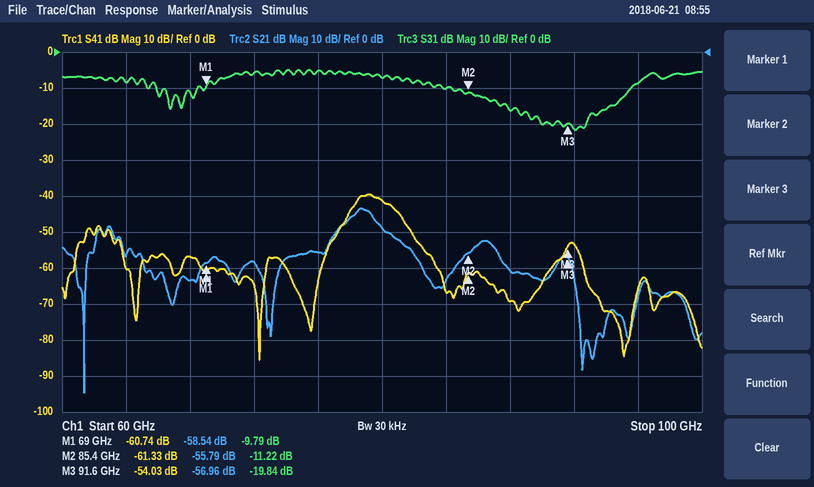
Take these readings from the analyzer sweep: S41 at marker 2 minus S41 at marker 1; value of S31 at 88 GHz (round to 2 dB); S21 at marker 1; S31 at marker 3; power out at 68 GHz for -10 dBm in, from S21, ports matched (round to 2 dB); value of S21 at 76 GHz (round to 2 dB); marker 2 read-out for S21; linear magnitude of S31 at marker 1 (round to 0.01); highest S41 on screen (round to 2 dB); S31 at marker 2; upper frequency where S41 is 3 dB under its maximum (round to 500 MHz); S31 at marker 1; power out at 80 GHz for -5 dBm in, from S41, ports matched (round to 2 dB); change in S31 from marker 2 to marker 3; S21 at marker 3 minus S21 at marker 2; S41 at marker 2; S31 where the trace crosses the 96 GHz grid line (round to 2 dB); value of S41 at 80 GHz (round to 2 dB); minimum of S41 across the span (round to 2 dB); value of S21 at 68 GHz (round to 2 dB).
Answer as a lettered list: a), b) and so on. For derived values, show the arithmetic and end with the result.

a) -61.33 − (-60.74) = -0.59 dB
b) -16 dB
c) -58.54 dB
d) -19.84 dB
e) -10 dBm + (-64 dB) = -74 dBm
f) -56 dB
g) -55.79 dB
h) 10^(-9.79/20) ≈ 0.32
i) -40 dB
j) -11.22 dB
k) 80.5 GHz
l) -9.79 dB
m) -5 dBm + (-42 dB) = -46 dBm
n) -19.84 − (-11.22) = -8.62 dB
o) -56.96 − (-55.79) = -1.17 dB
p) -61.33 dB
q) -8 dB
r) -42 dB
s) -86 dB
t) -64 dB
